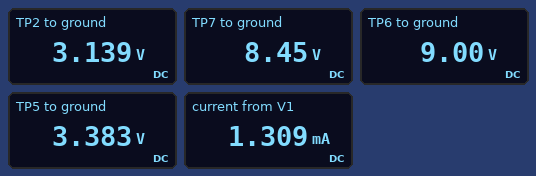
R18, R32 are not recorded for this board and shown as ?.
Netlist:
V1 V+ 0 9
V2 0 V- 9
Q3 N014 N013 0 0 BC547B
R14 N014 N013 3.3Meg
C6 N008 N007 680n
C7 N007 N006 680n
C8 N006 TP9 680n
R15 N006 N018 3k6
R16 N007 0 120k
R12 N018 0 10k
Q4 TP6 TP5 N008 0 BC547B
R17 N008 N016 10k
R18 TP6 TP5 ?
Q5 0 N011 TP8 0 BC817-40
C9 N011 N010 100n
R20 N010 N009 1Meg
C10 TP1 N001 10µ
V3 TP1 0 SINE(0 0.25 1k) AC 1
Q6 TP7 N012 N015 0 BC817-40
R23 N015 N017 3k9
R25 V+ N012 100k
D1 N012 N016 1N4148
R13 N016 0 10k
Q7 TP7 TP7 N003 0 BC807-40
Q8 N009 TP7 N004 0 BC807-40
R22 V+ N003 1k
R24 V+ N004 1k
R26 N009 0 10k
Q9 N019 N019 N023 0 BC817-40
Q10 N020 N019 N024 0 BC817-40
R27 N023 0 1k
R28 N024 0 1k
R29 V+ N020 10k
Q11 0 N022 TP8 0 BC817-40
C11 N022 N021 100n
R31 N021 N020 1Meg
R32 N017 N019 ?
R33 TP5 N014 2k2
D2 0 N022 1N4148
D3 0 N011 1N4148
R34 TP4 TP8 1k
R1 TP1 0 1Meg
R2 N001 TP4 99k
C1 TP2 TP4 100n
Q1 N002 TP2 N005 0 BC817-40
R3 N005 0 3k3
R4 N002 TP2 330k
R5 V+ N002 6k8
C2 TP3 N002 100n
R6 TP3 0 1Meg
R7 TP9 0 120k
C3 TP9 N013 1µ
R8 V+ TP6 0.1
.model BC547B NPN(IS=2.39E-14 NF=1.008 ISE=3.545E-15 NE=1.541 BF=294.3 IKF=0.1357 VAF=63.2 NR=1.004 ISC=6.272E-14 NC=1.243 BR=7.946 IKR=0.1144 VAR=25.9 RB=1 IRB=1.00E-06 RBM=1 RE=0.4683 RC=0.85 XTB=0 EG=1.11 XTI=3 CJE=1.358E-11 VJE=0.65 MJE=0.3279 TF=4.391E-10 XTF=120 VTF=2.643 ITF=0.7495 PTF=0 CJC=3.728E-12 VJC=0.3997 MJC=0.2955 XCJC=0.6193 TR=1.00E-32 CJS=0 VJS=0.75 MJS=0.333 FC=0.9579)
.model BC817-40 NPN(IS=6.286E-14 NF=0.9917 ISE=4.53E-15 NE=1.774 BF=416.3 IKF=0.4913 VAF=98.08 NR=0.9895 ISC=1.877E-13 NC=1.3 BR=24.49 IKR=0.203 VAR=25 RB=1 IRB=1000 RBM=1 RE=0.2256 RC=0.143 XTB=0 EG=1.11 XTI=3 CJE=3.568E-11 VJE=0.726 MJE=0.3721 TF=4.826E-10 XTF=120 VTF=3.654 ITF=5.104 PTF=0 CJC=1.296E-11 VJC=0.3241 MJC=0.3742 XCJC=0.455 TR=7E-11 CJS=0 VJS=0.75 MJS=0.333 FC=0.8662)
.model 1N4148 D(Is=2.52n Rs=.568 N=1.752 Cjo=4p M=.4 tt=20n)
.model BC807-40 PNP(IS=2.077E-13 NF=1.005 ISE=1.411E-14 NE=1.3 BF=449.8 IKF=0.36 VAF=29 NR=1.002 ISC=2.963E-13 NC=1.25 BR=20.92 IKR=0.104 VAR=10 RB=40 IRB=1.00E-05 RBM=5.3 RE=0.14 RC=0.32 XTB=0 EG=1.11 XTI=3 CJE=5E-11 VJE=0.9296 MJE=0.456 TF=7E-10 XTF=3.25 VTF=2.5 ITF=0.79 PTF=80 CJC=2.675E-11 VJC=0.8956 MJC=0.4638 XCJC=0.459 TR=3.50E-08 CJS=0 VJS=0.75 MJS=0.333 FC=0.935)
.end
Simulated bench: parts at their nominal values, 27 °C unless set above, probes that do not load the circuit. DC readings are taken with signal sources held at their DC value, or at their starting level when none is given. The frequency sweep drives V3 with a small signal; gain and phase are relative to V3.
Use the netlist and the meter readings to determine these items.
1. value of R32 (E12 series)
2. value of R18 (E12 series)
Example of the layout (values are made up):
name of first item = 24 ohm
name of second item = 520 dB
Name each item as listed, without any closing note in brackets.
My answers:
value of R32 = 18 kΩ
value of R18 = 27 kΩ
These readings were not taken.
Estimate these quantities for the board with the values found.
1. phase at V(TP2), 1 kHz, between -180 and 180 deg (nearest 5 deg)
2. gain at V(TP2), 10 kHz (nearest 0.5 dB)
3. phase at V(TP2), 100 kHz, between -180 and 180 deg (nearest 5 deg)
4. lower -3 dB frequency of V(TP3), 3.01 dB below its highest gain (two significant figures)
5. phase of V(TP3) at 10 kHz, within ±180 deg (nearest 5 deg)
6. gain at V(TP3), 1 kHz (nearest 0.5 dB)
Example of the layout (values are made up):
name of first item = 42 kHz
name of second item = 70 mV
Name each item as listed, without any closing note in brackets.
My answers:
phase at V(TP2), 1 kHz, between -180 and 180 deg = 0 deg
gain at V(TP2), 10 kHz = -6.5 dB
phase at V(TP2), 100 kHz, between -180 and 180 deg = -55 deg
lower -3 dB frequency of V(TP3), 3.01 dB below its highest gain = 8.3 Hz
phase of V(TP3) at 10 kHz, within ±180 deg = 170 deg
gain at V(TP3), 1 kHz = 0 dB
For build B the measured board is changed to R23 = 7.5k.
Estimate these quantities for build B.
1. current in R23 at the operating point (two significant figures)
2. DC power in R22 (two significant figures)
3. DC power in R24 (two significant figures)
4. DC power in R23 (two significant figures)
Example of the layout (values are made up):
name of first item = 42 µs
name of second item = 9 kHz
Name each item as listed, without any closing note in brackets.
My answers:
current in R23 at the operating point = 44 µA
DC power in R22 = 1.9 µW
DC power in R24 = 2.3 µW
DC power in R23 = 14 µW
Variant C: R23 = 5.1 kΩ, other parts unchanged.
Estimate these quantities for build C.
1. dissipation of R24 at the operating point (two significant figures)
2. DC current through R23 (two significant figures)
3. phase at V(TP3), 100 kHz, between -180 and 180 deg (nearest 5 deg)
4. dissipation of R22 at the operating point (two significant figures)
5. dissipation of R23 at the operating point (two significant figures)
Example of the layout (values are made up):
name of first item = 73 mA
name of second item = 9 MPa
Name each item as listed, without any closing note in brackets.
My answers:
dissipation of R24 at the operating point = 2.7 µW
DC current through R23 = 48 µA
phase at V(TP3), 100 kHz, between -180 and 180 deg = 120 deg
dissipation of R22 at the operating point = 2.3 µW
dissipation of R23 at the operating point = 12 µW
